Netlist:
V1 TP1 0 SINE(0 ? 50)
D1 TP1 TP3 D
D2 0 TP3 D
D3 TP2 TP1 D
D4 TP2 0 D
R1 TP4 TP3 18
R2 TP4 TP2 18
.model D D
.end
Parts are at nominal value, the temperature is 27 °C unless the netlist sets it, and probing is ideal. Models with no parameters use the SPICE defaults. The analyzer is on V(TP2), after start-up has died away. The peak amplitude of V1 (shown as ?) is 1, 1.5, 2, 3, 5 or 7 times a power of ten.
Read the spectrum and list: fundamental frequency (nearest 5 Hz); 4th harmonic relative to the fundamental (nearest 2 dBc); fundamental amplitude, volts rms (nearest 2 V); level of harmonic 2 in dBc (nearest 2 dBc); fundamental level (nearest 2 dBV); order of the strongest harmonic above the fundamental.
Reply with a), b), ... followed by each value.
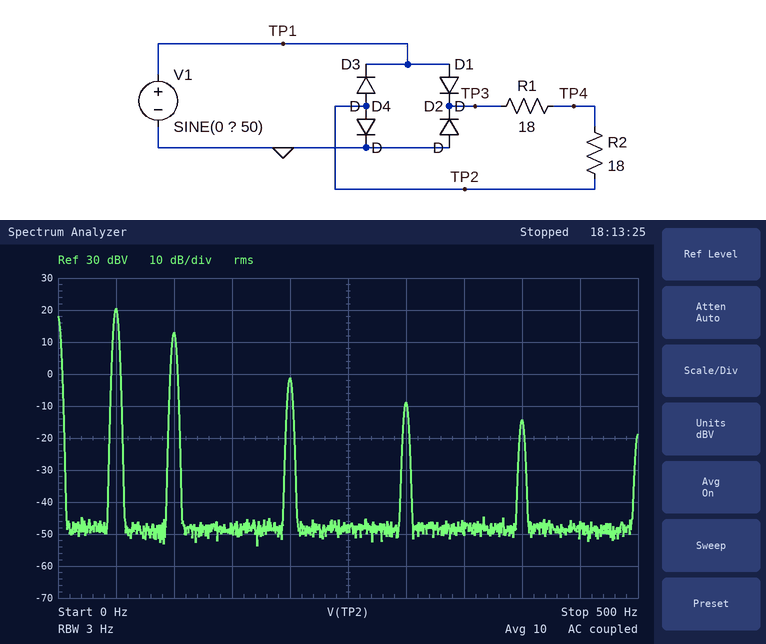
a) 50 Hz
b) -22 dBc
c) 10 V
d) -8 dBc
e) 20 dBV
f) 2
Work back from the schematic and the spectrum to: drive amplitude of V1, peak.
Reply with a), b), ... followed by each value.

a) 30 V
